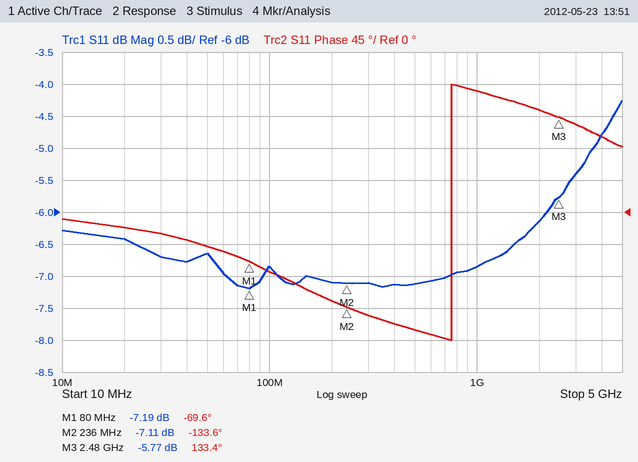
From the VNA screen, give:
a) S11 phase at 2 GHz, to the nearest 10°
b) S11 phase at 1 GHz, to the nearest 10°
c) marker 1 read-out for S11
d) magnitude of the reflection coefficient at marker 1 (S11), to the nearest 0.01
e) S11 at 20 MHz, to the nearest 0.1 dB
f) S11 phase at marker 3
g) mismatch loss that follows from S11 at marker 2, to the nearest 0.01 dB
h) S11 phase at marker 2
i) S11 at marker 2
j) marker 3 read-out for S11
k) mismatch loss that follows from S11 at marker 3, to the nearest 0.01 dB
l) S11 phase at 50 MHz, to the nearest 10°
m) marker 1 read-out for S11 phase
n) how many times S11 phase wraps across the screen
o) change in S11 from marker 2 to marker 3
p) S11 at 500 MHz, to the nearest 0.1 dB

140°
170°
-7.19 dB
0.44
-6.4 dB
133.4°
0.94 dB
-133.6°
-7.11 dB
-5.77 dB
1.34 dB
-50°
-69.6°
1
1.34 dB
-7.1 dB
